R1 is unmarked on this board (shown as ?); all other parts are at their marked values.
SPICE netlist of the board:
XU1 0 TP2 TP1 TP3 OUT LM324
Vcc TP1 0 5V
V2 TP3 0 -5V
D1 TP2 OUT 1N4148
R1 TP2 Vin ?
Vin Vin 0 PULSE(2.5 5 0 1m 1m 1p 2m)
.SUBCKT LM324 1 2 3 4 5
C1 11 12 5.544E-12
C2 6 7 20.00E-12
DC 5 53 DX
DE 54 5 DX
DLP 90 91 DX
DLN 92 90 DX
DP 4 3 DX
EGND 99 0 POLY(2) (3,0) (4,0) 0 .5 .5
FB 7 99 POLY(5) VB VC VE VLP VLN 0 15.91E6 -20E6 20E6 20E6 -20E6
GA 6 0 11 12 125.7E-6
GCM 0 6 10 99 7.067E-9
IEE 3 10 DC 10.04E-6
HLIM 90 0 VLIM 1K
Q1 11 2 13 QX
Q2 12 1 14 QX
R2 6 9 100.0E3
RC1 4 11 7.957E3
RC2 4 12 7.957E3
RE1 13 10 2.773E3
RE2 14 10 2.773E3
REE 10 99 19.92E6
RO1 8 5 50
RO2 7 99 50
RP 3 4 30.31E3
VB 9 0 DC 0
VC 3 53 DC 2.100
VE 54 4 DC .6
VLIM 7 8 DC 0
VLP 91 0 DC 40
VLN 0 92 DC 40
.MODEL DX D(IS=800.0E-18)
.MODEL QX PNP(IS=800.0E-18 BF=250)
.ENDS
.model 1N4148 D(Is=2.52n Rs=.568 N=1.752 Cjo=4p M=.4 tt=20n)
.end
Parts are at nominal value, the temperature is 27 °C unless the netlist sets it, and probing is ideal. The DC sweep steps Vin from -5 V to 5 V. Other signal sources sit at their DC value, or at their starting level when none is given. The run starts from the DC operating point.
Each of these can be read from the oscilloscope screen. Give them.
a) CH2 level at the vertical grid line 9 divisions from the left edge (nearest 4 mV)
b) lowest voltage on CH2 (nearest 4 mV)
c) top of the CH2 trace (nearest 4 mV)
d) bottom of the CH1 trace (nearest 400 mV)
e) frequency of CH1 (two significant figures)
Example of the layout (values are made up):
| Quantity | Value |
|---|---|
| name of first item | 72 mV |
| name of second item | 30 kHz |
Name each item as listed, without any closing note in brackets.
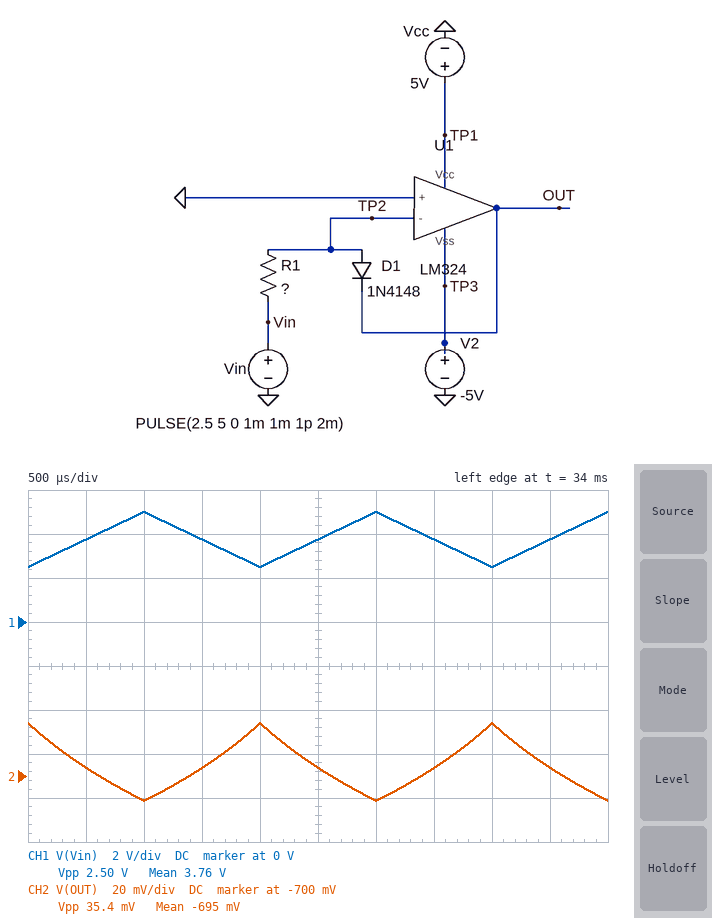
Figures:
| Quantity | Value |
|---|---|
| CH2 level at the vertical grid line 9 divisions from the left edge | -696 mV |
| lowest voltage on CH2 | -712 mV |
| top of the CH2 trace | -676 mV |
| bottom of the CH1 trace | 2.4 V |
| frequency of CH1 | 500 Hz |
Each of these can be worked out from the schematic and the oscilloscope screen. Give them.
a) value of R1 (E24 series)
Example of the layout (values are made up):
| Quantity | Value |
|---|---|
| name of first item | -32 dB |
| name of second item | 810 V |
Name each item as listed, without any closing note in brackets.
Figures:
| Quantity | Value |
|---|---|
| value of R1 | 360 Ω |
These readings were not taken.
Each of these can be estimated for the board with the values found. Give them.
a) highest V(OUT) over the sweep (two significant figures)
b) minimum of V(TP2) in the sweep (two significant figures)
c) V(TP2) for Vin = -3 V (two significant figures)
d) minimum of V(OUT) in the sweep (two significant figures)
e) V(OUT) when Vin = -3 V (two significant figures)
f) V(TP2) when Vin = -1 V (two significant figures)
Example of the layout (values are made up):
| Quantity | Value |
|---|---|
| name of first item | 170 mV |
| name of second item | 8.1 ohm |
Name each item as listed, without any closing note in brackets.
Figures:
| Quantity | Value |
|---|---|
| highest V(OUT) over the sweep | 3.5 V |
| minimum of V(TP2) in the sweep | -5.0 V |
| V(TP2) for Vin = -3 V | -3.0 V |
| minimum of V(OUT) in the sweep | -710 mV |
| V(OUT) when Vin = -3 V | 3.5 V |
| V(TP2) when Vin = -1 V | -1.0 V |
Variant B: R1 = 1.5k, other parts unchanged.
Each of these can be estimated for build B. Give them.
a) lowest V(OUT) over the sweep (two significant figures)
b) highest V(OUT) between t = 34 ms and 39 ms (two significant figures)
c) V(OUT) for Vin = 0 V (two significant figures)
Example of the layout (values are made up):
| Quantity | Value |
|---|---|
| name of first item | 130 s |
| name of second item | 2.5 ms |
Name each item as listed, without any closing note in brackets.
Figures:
| Quantity | Value |
|---|---|
| lowest V(OUT) over the sweep | -640 mV |
| highest V(OUT) between t = 34 ms and 39 ms | -610 mV |
| V(OUT) for Vin = 0 V | -130 mV |
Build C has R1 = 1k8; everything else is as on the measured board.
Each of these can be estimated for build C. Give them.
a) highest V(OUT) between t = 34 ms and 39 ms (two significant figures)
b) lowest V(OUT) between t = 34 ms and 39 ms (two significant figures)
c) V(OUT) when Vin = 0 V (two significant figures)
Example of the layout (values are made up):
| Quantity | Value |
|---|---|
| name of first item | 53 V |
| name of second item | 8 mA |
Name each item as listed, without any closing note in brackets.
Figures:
| Quantity | Value |
|---|---|
| highest V(OUT) between t = 34 ms and 39 ms | -600 mV |
| lowest V(OUT) between t = 34 ms and 39 ms | -630 mV |
| V(OUT) when Vin = 0 V | -130 mV |
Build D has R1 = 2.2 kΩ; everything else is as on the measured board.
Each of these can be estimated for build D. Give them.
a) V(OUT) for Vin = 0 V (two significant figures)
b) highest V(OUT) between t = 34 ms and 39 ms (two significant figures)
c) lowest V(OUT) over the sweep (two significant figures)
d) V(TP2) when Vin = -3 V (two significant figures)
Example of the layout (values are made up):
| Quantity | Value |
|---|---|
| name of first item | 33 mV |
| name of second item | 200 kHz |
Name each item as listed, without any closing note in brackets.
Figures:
| Quantity | Value |
|---|---|
| V(OUT) for Vin = 0 V | -120 mV |
| highest V(OUT) between t = 34 ms and 39 ms | -590 mV |
| lowest V(OUT) over the sweep | -620 mV |
| V(TP2) when Vin = -3 V | -3.0 V |
